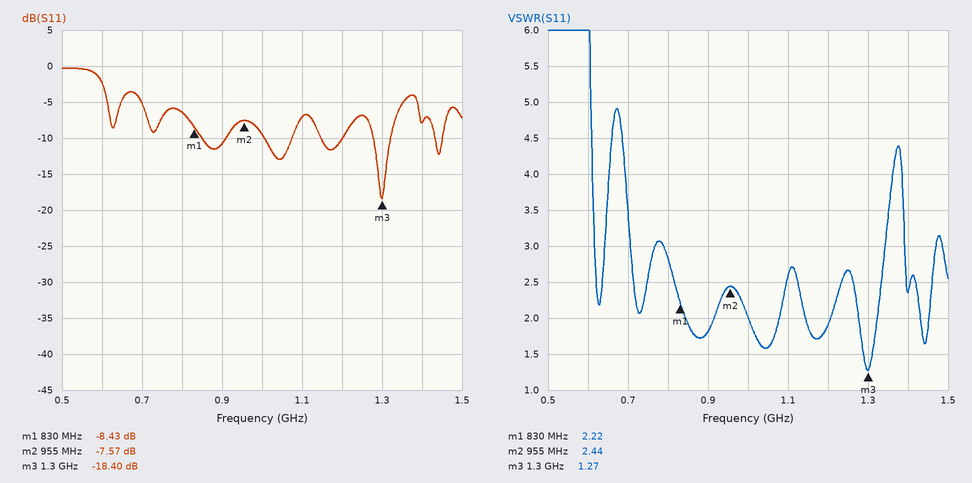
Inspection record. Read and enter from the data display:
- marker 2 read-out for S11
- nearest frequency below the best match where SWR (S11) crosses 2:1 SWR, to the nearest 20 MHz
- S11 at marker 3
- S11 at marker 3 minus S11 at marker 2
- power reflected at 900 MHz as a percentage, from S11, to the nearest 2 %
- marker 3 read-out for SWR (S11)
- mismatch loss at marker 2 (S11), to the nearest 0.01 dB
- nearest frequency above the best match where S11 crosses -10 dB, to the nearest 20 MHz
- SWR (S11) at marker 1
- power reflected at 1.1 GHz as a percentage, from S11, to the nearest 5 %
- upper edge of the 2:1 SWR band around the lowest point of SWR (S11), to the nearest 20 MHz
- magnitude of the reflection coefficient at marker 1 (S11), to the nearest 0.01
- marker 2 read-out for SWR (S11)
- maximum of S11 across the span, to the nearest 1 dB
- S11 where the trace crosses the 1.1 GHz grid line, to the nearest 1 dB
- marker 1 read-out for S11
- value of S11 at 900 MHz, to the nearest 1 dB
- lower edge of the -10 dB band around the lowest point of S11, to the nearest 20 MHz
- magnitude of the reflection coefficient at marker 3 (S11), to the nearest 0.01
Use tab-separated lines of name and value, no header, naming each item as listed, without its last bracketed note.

marker 2 read-out for S11	-7.57 dB
nearest frequency below the best match where SWR (S11) crosses 2:1 SWR, to the nearest 20 MHz	1.28 GHz
S11 at marker 3	-18.40 dB
S11 at marker 3 minus S11 at marker 2	-10.83 dB
power reflected at 900 MHz as a percentage, from S11, to the nearest 2 %	8 %
marker 3 read-out for SWR	1.27
mismatch loss at marker 2 (S11), to the nearest 0.01 dB	0.84 dB
nearest frequency above the best match where S11 crosses -10 dB, to the nearest 20 MHz	1.32 GHz
SWR (S11) at marker 1	2.22
power reflected at 1.1 GHz as a percentage, from S11, to the nearest 5 %	20 %
upper edge of the 2:1 SWR band around the lowest point of SWR (S11), to the nearest 20 MHz	1.32 GHz
magnitude of the reflection coefficient at marker 1 (S11), to the nearest 0.01	0.38
marker 2 read-out for SWR	2.44
maximum of S11 across the span, to the nearest 1 dB	0 dB
S11 where the trace crosses the 1.1 GHz grid line, to the nearest 1 dB	-7 dB
marker 1 read-out for S11	-8.43 dB
value of S11 at 900 MHz, to the nearest 1 dB	-11 dB
lower edge of the -10 dB band around the lowest point of S11, to the nearest 20 MHz	1.28 GHz
magnitude of the reflection coefficient at marker 3 (S11), to the nearest 0.01	0.12
